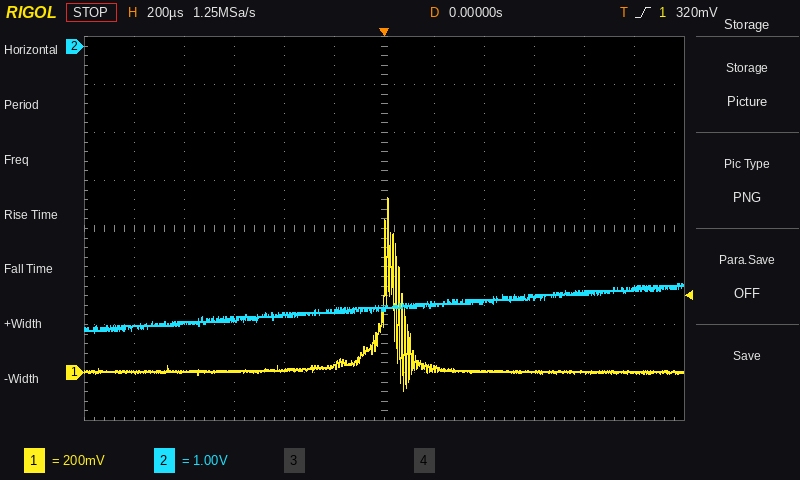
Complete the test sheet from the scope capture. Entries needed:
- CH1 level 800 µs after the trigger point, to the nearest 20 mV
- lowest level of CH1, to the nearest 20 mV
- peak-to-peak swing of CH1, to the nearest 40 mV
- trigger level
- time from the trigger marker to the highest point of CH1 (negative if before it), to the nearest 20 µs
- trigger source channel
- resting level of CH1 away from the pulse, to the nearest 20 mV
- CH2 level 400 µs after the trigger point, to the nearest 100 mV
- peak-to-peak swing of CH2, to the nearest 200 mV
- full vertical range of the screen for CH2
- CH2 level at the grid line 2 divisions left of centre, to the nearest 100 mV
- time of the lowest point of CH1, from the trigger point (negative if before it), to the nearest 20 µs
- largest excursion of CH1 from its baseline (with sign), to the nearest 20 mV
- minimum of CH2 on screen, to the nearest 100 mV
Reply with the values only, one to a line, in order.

0 mV
-80 mV
800 mV
320 mV
+20 µs
CH1
0 mV
-5.3 V
1.0 V
8 V
-5.6 V
+80 µs
+720 mV
-6.0 V
